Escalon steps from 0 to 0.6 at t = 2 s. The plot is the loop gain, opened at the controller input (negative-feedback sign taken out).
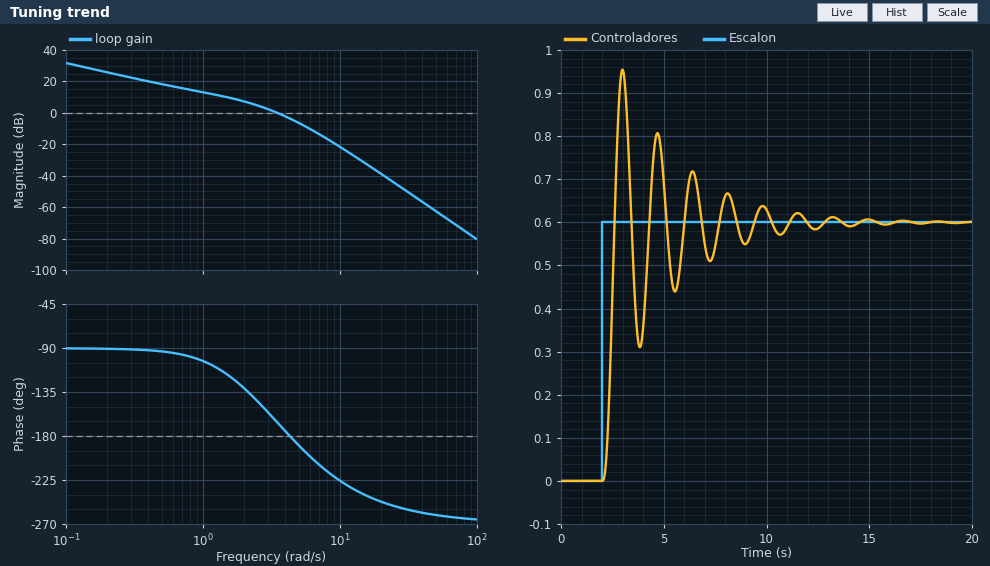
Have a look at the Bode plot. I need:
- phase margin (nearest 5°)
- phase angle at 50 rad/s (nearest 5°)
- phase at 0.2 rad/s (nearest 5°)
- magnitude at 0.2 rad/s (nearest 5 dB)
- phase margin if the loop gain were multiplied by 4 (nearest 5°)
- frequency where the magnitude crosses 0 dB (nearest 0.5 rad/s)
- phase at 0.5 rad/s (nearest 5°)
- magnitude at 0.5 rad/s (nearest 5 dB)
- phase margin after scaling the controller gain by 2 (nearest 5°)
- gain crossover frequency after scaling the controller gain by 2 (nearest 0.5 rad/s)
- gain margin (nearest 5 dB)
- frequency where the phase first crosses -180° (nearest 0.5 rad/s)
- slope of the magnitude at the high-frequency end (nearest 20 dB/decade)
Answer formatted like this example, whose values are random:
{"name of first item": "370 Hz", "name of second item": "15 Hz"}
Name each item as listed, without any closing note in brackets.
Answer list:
{"phase margin": "15°", "phase angle at 50 rad/s": "-260°", "phase at 0.2 rad/s": "-90°", "magnitude at 0.2 rad/s": "25 dB", "phase margin if the loop gain were multiplied by 4": "-25°", "frequency where the magnitude crosses 0 dB": "3.5 rad/s", "phase at 0.5 rad/s": "-95°", "magnitude at 0.5 rad/s": "20 dB", "phase margin after scaling the controller gain by 2": "-10°", "gain crossover frequency after scaling the controller gain by 2": "5.0 rad/s", "gain margin": "5 dB", "frequency where the phase first crosses -180°": "4.5 rad/s", "slope of the magnitude at the high-frequency end": "-60 dB/decade"}
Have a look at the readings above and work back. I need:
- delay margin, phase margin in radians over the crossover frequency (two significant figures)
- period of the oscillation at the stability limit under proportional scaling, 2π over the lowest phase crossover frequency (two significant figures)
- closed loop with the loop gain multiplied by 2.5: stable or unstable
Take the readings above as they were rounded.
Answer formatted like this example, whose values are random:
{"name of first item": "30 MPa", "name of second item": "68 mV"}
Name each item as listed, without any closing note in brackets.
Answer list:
{"delay margin, phase margin in radians over the crossover frequency": "0.075 s", "period of the oscillation at the stability limit under proportional scaling, 2π over the lowest phase crossover frequency": "1.4 s", "closed loop with the loop gain multiplied by 2.5: stable or unstable": "unstable"}
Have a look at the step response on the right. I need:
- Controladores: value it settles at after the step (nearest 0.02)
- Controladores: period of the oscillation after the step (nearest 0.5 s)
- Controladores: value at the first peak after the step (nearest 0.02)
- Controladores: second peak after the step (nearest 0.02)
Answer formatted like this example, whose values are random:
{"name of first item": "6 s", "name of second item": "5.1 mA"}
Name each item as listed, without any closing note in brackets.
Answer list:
{"Controladores: value it settles at after the step": "0.60", "Controladores: period of the oscillation after the step": "1.5 s", "Controladores: value at the first peak after the step": "0.96", "Controladores: second peak after the step": "0.80"}
